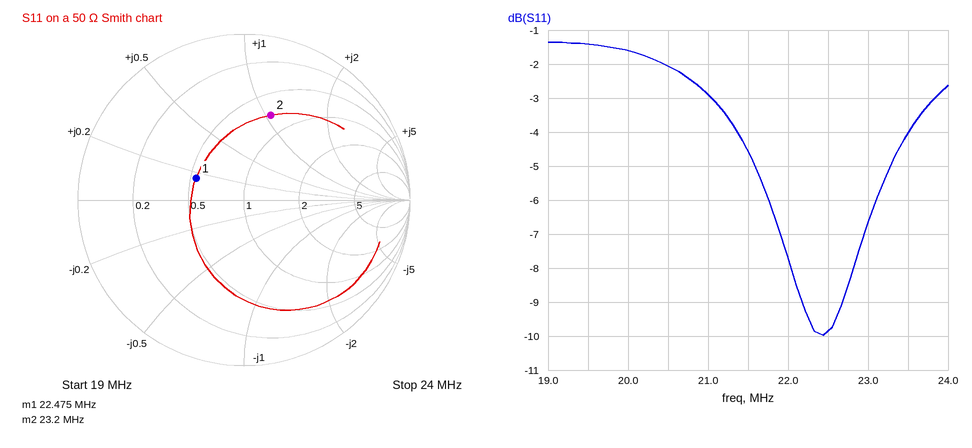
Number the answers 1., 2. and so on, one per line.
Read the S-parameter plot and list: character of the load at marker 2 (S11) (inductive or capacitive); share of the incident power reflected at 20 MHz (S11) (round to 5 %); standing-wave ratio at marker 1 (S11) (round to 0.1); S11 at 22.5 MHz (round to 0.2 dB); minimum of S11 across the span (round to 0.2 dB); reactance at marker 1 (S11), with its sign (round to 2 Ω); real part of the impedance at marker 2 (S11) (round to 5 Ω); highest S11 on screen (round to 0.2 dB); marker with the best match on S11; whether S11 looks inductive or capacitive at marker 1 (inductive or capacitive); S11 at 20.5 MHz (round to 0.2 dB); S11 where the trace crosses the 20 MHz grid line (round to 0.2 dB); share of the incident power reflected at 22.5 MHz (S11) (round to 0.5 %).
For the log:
1. inductive
2. 70 %
3. 1.9
4. -9.8 dB
5. -10.0 dB
6. +8 Ω
7. 35 Ω
8. -1.4 dB
9. marker 1
10. inductive
11. -2.0 dB
12. -1.6 dB
13. 10.5 %
